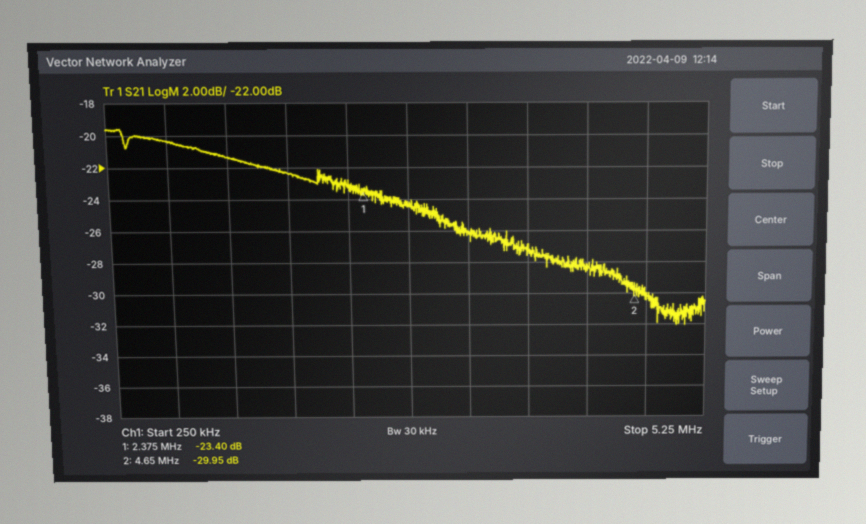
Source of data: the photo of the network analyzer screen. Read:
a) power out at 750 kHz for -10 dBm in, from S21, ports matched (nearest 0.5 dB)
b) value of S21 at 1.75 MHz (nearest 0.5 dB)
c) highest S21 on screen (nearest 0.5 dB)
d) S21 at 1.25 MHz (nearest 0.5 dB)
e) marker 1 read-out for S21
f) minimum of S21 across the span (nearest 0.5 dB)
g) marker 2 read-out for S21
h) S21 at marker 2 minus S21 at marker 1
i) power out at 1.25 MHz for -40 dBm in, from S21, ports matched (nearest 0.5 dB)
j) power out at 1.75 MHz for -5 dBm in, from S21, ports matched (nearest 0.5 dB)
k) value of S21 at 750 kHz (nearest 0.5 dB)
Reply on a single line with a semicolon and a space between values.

-30.5 dBm; -22.5 dB; -19.5 dB; -21.5 dB; -23.40 dB; -32.0 dB; -29.95 dB; -6.55 dB; -61.5 dBm; -27.5 dBm; -20.5 dB
